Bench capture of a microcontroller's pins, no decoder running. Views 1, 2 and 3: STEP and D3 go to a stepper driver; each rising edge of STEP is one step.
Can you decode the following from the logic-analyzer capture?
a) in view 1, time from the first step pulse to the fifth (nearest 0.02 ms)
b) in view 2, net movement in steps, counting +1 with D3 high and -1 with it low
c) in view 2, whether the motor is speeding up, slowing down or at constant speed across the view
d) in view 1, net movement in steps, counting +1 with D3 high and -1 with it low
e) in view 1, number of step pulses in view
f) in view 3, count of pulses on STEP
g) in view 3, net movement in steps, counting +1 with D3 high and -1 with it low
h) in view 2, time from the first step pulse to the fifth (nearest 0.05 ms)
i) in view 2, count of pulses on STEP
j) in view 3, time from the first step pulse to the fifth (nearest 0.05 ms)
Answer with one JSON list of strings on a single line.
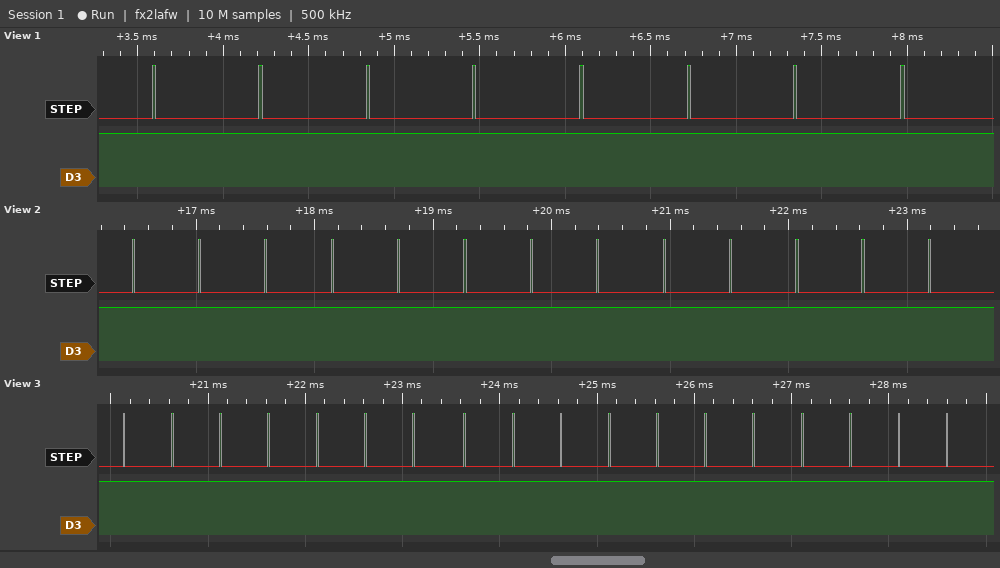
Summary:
["2.50 ms", "+13", "constant speed", "+8", "8", "18", "+18", "2.25 ms", "13", "2.00 ms"]
